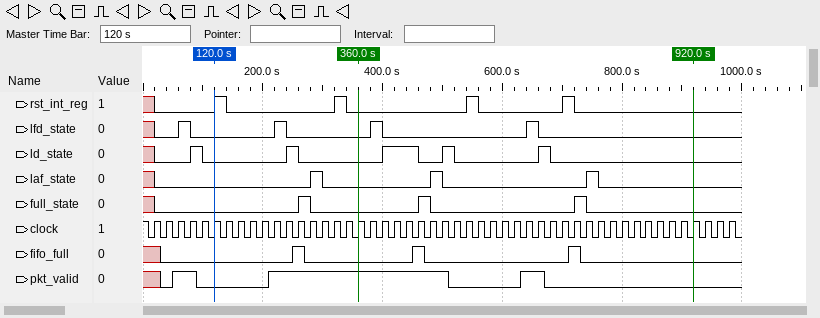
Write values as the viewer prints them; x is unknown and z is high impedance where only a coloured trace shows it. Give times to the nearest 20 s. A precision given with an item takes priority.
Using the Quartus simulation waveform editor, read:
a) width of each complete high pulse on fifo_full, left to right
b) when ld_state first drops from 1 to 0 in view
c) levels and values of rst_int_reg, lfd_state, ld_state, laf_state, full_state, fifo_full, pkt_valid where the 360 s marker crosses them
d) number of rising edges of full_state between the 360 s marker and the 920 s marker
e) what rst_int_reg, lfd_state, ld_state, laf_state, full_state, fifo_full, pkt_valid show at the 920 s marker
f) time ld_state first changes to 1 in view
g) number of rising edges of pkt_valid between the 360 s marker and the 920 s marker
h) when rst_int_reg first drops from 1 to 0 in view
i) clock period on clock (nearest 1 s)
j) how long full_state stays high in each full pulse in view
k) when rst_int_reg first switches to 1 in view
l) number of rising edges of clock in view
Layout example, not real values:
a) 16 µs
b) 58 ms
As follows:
a) 20 s, 20 s, 20 s
b) 100 s
c) rst_int_reg=0, lfd_state=0, ld_state=0, laf_state=0, full_state=0, fifo_full=0, pkt_valid=1
d) 2
e) rst_int_reg=0, lfd_state=0, ld_state=0, laf_state=0, full_state=0, fifo_full=0, pkt_valid=0
f) 80 s
g) 1
h) 140 s
i) 20 s
j) 20 s, 20 s, 20 s
k) 120 s
l) 49
